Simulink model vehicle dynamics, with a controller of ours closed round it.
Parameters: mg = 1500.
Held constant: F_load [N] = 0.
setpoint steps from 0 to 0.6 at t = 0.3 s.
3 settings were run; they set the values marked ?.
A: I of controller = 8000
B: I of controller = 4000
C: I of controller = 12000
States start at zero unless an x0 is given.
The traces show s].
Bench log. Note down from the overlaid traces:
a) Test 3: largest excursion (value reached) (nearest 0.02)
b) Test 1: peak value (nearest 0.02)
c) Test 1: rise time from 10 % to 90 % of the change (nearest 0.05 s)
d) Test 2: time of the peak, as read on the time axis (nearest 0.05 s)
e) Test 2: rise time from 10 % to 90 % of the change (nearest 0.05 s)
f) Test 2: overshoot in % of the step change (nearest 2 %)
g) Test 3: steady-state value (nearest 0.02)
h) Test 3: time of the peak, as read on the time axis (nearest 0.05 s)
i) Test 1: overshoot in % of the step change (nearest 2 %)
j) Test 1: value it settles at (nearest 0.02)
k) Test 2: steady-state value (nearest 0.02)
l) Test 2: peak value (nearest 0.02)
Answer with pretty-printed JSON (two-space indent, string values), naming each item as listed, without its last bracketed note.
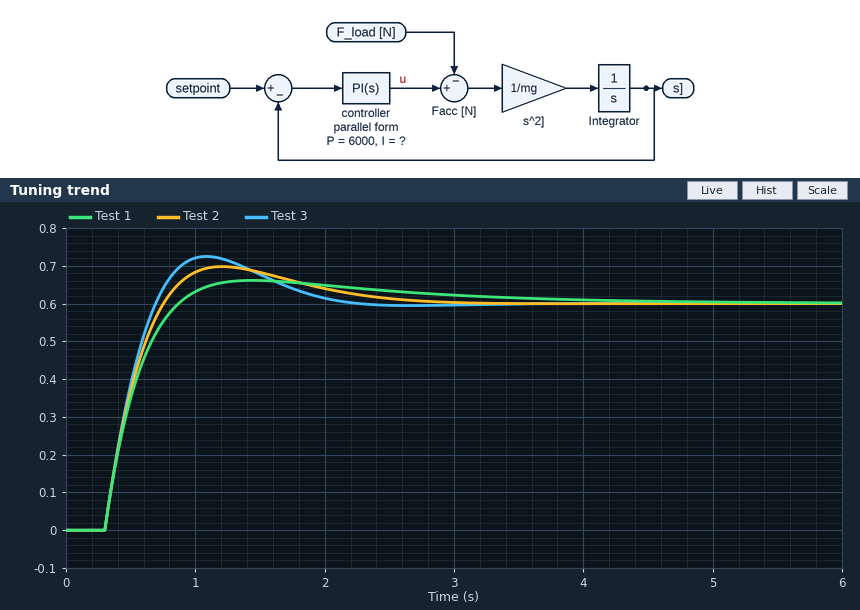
{
  "Test 3: largest excursion (value reached)": "0.72",
  "Test 1: peak value": "0.66",
  "Test 1: rise time from 10 % to 90 % of the change": "0.40 s",
  "Test 2: time of the peak, as read on the time axis": "1.20 s",
  "Test 2: rise time from 10 % to 90 % of the change": "0.35 s",
  "Test 2: overshoot in % of the step change": "16 %",
  "Test 3: steady-state value": "0.60",
  "Test 3: time of the peak, as read on the time axis": "1.10 s",
  "Test 1: overshoot in % of the step change": "10 %",
  "Test 1: value it settles at": "0.60",
  "Test 2: steady-state value": "0.60",
  "Test 2: peak value": "0.70"
}
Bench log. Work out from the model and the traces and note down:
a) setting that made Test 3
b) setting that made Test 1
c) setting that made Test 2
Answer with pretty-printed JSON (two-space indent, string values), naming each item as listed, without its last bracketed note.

{
  "setting that made Test 3": "C",
  "setting that made Test 1": "B",
  "setting that made Test 2": "A"
}
